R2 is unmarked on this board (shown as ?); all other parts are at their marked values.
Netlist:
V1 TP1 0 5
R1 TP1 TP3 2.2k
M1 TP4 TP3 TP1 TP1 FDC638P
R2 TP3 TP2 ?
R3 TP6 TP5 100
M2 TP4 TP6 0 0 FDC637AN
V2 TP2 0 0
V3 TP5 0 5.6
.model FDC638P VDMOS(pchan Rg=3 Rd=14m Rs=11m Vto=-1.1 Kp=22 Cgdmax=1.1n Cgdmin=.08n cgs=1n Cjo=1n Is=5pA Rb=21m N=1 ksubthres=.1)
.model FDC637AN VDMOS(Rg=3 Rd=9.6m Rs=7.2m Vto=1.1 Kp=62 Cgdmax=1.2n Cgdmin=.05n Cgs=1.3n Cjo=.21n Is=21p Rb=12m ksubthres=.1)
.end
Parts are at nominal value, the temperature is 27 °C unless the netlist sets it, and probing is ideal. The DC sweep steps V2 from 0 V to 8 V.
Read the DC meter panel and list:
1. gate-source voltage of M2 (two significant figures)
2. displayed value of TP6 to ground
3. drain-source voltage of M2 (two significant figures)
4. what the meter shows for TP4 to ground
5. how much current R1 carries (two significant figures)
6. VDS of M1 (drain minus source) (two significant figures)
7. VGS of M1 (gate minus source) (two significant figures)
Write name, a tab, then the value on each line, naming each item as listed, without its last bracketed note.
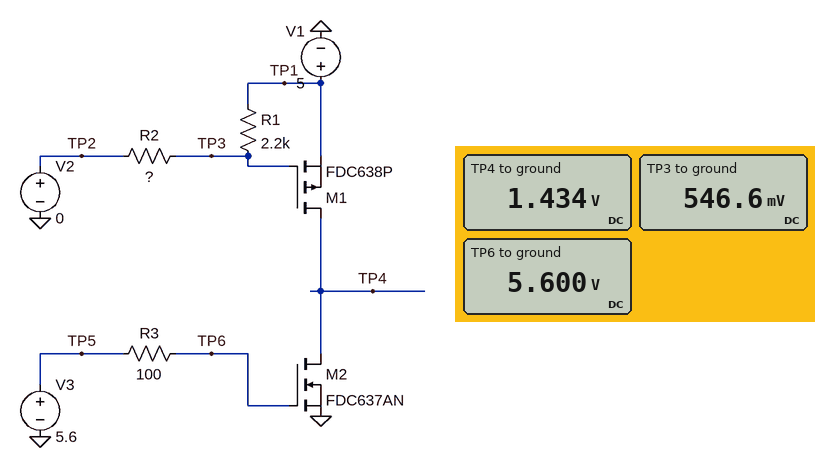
gate-source voltage of M2	5.6 V
displayed value of TP6 to ground	5.600 V
drain-source voltage of M2	1.4 V
what the meter shows for TP4 to ground	1.434 V
how much current R1 carries	2.0 mA
VDS of M1 (drain minus source)	-3.6 V
VGS of M1 (gate minus source)	-4.5 V
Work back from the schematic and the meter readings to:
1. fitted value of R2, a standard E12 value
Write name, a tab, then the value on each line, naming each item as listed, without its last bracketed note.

fitted value of R2, a standard E12 value	270 Ω
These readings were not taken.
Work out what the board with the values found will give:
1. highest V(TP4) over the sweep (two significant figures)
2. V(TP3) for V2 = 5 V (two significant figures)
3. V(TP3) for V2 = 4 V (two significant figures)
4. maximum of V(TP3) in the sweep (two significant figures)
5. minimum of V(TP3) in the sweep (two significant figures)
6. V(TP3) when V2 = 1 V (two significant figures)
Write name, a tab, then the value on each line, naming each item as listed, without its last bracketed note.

highest V(TP4) over the sweep	1.4 V
V(TP3) for V2 = 5 V	5.0 V
V(TP3) for V2 = 4 V	4.1 V
maximum of V(TP3) in the sweep	7.7 V
minimum of V(TP3) in the sweep	550 mV
V(TP3) when V2 = 1 V	1.4 V
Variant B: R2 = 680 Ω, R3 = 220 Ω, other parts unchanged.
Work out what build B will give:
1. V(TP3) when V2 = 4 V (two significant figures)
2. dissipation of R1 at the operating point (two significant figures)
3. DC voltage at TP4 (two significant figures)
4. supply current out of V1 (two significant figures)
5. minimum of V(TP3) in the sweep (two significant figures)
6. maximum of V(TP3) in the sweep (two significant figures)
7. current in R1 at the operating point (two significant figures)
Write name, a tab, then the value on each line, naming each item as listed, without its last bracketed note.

V(TP3) when V2 = 4 V	4.2 V
dissipation of R1 at the operating point	6.6 mW
DC voltage at TP4	1.1 V
supply current out of V1	51 A
minimum of V(TP3) in the sweep	1.2 V
maximum of V(TP3) in the sweep	7.3 V
current in R1 at the operating point	1.7 mA
